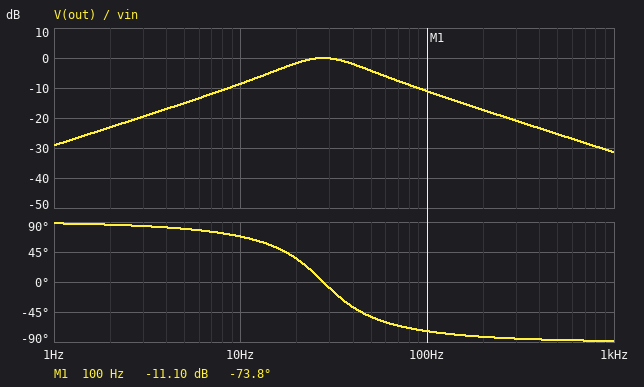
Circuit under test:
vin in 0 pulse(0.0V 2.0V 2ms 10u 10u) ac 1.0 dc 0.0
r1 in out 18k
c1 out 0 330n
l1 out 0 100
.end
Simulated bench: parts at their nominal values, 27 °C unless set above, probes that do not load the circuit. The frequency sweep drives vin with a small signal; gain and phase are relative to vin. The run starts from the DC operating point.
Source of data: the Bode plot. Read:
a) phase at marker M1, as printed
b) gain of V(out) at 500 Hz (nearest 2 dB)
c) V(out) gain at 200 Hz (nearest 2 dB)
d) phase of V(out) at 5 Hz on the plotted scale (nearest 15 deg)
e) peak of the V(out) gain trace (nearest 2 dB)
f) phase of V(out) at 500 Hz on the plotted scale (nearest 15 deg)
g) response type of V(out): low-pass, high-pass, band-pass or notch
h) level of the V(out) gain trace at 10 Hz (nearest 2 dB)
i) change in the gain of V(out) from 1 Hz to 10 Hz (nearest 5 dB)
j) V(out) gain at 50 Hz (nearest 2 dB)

-73.8 deg
-26 dB
-18 dB
75 deg
0 dB
-90 deg
band-pass
-8 dB
20 dB
-4 dB
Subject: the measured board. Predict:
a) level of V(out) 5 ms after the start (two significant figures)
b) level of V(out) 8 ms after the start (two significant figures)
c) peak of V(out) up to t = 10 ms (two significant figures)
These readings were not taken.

760 mV
1.1 V
1.1 V
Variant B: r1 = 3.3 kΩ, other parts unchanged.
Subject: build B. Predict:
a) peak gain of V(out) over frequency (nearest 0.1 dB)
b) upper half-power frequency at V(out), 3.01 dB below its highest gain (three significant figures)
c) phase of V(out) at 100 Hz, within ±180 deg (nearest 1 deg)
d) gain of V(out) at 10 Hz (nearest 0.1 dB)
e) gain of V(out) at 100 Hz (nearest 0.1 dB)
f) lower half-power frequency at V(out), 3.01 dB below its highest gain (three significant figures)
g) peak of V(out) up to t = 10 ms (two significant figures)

0 dB
151 Hz
-32 deg
-0.8 dB
-1.5 dB
5.08 Hz
1.8 V
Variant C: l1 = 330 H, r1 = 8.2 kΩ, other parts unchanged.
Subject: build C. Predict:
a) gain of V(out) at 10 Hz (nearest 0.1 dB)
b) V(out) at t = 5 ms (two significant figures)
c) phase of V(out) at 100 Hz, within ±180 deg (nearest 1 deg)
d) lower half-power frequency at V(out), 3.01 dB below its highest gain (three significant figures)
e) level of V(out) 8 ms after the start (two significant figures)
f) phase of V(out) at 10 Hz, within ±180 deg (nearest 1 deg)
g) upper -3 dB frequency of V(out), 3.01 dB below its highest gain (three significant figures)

-0.2 dB
1.3 V
-59 deg
3.72 Hz
1.7 V
13 deg
62.5 Hz
